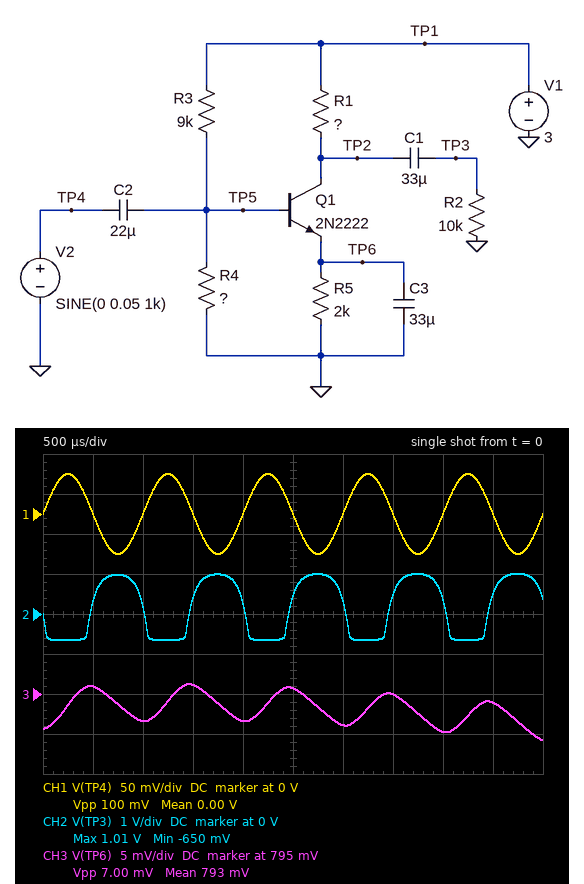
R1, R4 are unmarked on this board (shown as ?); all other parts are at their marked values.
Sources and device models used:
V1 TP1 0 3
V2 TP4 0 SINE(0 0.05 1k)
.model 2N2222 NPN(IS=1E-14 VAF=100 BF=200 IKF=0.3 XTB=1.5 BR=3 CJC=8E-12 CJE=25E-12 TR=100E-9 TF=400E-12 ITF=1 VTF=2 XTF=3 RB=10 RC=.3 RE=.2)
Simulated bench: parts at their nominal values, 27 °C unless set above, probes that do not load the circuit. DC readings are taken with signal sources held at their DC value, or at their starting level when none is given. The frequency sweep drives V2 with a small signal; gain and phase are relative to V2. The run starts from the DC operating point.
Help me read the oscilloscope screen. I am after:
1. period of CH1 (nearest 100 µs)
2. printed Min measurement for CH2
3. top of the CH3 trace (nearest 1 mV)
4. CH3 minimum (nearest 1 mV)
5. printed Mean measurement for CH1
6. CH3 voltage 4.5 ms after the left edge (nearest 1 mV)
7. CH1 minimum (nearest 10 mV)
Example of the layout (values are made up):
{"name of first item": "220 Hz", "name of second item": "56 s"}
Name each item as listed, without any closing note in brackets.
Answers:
{"period of CH1": "1.0 ms", "printed Min measurement for CH2": "-650 mV", "top of the CH3 trace": "796 mV", "CH3 minimum": "789 mV", "printed Mean measurement for CH1": "0.00 V", "CH3 voltage 4.5 ms after the left edge": "794 mV", "CH1 minimum": "-50 mV"}
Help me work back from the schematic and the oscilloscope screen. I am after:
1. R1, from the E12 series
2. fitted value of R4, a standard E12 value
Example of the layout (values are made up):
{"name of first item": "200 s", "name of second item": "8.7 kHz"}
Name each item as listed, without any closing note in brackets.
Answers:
{"R1, from the E12 series": "3.9 kΩ", "fitted value of R4, a standard E12 value": "8.2 kΩ"}
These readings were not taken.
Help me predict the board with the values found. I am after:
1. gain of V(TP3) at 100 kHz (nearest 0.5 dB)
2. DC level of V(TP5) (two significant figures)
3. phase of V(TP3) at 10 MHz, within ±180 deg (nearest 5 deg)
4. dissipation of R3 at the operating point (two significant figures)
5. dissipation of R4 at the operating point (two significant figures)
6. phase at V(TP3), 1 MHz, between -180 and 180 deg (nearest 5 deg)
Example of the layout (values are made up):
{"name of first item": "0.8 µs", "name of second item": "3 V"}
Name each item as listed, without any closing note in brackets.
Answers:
{"gain of V(TP3) at 100 kHz": "32.5 dB", "DC level of V(TP5)": "1.4 V", "phase of V(TP3) at 10 MHz, within ±180 deg": "120 deg", "dissipation of R3 at the operating point": "280 µW", "dissipation of R4 at the operating point": "250 µW", "phase at V(TP3), 1 MHz, between -180 and 180 deg": "170 deg"}
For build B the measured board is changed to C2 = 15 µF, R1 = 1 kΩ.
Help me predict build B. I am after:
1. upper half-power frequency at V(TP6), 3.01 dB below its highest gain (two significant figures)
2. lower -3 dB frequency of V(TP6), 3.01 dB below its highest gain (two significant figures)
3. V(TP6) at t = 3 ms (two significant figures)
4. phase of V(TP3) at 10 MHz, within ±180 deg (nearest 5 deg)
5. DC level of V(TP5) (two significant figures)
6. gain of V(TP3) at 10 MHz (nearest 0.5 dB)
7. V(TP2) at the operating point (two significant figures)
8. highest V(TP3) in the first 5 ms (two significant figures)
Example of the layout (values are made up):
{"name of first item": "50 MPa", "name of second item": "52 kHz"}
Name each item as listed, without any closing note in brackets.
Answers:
{"upper half-power frequency at V(TP6), 3.01 dB below its highest gain": "81 Hz", "lower -3 dB frequency of V(TP6), 3.01 dB below its highest gain": "2.3 Hz", "V(TP6) at t = 3 ms": "800 mV", "phase of V(TP3) at 10 MHz, within ±180 deg": "155 deg", "DC level of V(TP5)": "1.4 V", "gain of V(TP3) at 10 MHz": "22.0 dB", "V(TP2) at the operating point": "2.6 V", "highest V(TP3) in the first 5 ms": "330 mV"}
